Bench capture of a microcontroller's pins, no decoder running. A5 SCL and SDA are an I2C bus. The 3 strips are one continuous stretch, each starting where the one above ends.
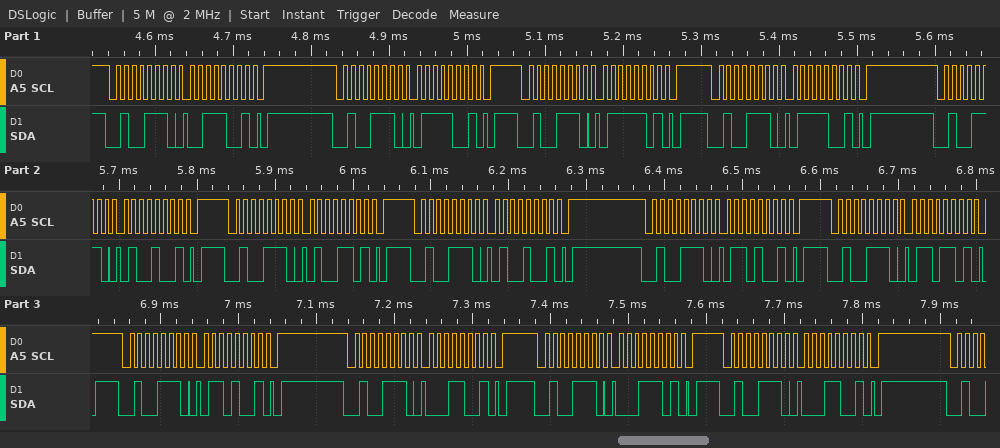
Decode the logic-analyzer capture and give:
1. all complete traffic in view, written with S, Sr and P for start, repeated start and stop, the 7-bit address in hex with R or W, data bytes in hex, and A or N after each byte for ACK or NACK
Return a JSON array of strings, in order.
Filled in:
["S 27W A 39 A P S 27W A 79 A P S 27W A 7D A P S 27W A 79 A P S 27W A 49 A P S 27W A 4D A P S 27W A 49 A P S 27W A 69 A P S 27W A 6D A P S 27W A 69 A P S 27W A 19 A P S 27W A 1D A P S 27W A 19 A P"]
